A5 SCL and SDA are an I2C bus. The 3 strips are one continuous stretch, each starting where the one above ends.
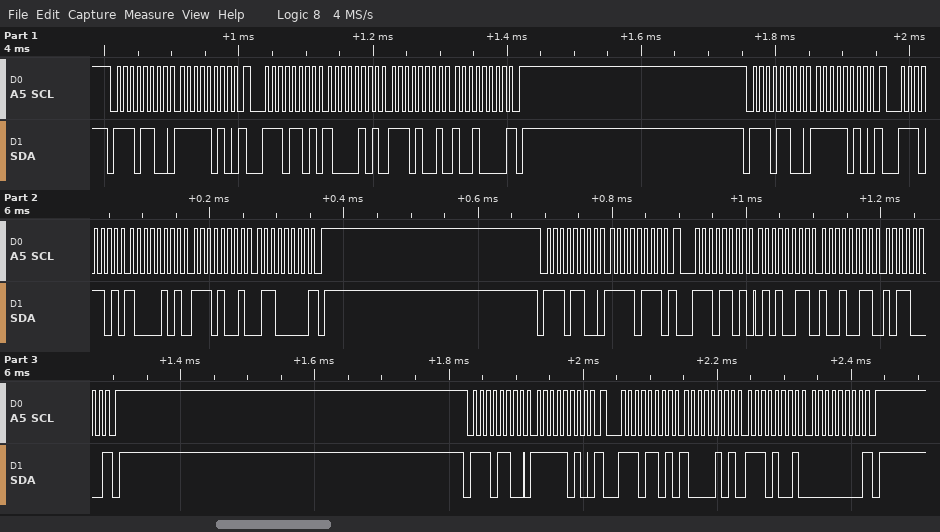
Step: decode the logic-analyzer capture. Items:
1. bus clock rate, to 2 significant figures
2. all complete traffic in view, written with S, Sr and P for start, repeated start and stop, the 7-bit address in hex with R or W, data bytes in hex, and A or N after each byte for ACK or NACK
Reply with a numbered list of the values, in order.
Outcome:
1. 100 kHz
2. S 76W A FA A Sr 76R A 85 A E9 A 90 N P S 76W A FA A Sr 76R A 85 A E9 A 60 N P S 76W A F7 A Sr 76R A 53 A 93 A B0 N P S 76W A FA A Sr 76R A 85 A E9 A 00 N P
